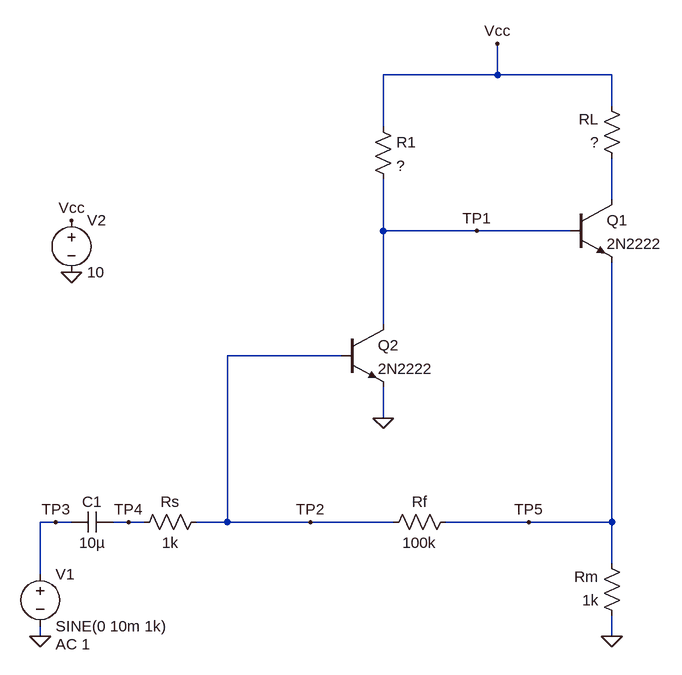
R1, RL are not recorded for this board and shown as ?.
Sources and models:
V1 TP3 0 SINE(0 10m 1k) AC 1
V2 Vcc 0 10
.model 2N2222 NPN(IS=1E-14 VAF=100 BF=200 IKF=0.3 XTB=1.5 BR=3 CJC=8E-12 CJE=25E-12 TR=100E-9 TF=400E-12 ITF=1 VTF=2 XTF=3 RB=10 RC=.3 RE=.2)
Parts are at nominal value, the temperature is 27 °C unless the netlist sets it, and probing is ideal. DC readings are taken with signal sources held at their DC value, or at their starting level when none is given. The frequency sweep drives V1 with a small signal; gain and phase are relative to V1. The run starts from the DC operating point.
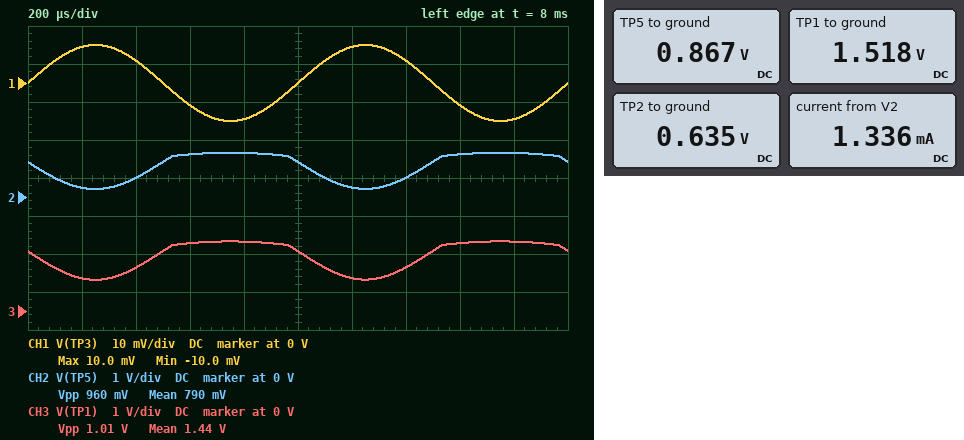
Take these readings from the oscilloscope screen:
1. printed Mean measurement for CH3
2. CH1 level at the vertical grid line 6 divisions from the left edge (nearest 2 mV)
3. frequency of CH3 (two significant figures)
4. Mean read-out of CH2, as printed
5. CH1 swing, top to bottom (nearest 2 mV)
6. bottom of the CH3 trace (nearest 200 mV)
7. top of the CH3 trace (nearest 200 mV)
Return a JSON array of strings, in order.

["1.44 V", "10 mV", "1.0 kHz", "790 mV", "20 mV", "800 mV", "1.8 V"]
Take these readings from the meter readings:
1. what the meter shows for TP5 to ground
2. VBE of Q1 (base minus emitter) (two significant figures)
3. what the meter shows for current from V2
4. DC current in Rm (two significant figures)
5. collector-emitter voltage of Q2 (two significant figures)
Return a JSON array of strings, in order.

["0.867 V", "650 mV", "1.336 mA", "870 µA", "1.5 V"]
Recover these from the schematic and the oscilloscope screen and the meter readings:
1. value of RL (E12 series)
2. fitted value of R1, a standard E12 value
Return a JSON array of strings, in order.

["8.2 kΩ", "18 kΩ"]
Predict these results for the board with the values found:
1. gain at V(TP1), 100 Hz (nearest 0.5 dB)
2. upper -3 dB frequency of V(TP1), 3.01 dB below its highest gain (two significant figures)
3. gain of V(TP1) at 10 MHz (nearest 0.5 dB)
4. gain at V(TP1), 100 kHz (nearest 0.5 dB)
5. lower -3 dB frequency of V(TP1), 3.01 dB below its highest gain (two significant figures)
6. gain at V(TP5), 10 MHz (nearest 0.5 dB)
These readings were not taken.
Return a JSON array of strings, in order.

["37.0 dB", "220 kHz", "4.0 dB", "36.5 dB", "12 Hz", "3.5 dB"]
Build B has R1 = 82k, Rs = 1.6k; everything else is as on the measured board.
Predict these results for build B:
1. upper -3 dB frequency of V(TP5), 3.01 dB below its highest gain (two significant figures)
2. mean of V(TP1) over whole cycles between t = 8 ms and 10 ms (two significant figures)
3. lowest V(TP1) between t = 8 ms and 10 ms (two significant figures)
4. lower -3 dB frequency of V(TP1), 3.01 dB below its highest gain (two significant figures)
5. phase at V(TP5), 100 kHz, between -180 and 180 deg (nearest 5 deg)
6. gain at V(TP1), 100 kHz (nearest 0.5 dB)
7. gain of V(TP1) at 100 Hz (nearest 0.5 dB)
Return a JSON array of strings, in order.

["140 kHz", "1.3 V", "780 mV", "7.7 Hz", "145 deg", "32.0 dB", "34.0 dB"]
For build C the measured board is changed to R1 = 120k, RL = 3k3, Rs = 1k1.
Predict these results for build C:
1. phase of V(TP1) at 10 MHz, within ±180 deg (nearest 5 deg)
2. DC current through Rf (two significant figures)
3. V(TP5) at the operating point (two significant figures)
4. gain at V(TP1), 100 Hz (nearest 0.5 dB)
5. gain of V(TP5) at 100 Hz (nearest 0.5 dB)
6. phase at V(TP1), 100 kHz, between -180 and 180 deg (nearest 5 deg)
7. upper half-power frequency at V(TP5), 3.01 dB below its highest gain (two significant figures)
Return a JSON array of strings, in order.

["50 deg", "350 nA", "620 mV", "36.0 dB", "35.5 dB", "145 deg", "150 kHz"]
